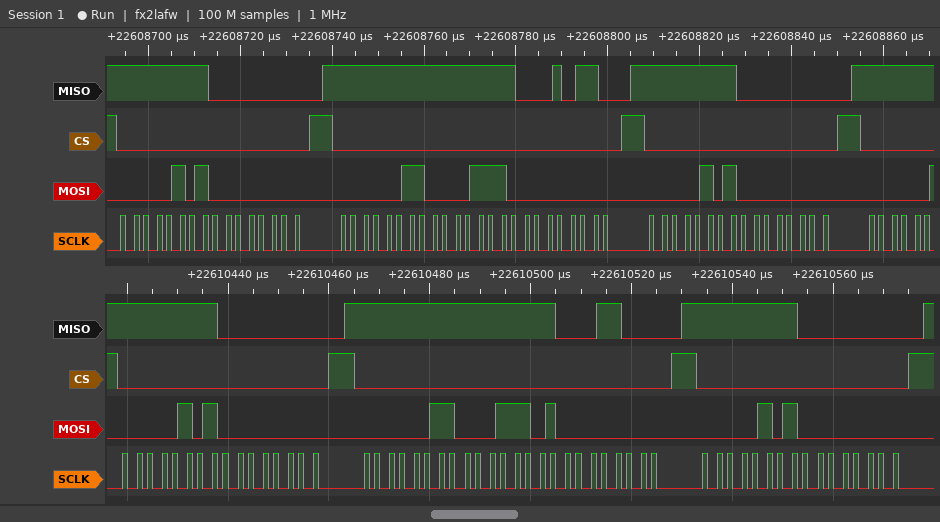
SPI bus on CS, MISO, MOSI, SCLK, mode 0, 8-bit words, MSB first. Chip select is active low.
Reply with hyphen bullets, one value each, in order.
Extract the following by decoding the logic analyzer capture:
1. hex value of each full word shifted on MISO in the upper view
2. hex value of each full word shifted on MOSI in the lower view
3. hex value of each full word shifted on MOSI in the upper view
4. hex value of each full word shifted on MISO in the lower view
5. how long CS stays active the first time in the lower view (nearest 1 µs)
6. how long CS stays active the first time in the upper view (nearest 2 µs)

- FF, 00, FF, FF, 16, FF, 00
- 05, 00, 03, 1D, 00, 05, 00
- 05, 00, 03, 0E, 00, 05, 00
- FF, 00, FF, FF, 18, FF, 00
- 42 µs
- 42 µs
